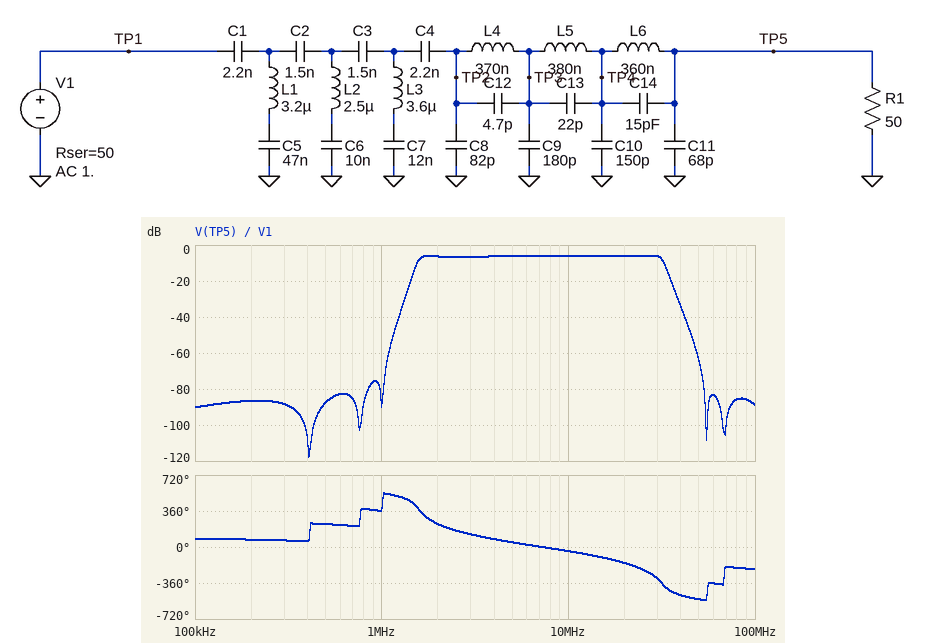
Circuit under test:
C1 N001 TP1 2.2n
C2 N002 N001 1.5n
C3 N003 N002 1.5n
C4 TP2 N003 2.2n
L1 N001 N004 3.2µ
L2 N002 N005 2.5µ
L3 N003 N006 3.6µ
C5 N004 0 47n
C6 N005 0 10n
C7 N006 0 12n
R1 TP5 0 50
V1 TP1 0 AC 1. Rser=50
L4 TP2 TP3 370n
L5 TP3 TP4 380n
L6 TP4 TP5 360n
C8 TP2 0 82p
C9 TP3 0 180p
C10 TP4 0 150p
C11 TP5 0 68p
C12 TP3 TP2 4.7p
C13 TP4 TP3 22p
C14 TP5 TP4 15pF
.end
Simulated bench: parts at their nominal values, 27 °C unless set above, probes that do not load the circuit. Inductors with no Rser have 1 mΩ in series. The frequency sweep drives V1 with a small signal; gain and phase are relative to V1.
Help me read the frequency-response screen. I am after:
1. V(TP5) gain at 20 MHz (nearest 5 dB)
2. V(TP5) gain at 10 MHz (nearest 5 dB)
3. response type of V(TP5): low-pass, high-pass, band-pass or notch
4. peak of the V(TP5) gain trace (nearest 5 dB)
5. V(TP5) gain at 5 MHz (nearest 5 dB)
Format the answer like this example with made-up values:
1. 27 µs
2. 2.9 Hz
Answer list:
1. -5 dB
2. -5 dB
3. band-pass
4. -5 dB
5. -5 dB
